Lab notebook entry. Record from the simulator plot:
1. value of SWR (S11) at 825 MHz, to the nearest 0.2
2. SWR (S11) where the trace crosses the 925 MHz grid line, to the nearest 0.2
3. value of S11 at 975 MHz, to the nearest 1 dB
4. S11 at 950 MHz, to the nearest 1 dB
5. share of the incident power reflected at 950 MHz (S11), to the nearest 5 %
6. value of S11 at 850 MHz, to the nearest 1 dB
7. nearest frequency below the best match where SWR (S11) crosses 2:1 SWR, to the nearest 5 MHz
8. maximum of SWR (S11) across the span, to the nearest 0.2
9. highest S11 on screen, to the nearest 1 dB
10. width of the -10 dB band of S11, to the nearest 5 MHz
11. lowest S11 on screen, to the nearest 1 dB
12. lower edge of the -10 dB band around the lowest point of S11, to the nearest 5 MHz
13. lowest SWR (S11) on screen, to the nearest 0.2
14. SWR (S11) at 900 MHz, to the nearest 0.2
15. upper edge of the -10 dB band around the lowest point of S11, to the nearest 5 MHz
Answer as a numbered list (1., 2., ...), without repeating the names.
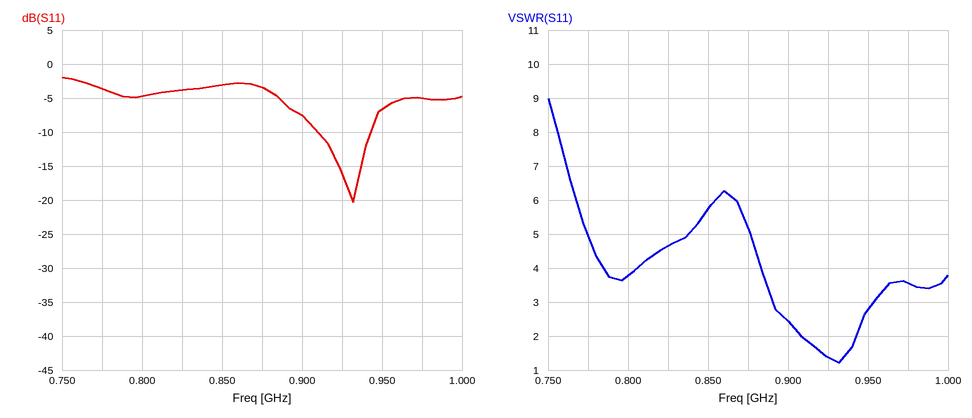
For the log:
1. 4.6
2. 1.4
3. -5 dB
4. -7 dB
5. 20 %
6. -3 dB
7. 910 MHz
8. 9.0
9. -2 dB
10. 35 MHz
11. -20 dB
12. 910 MHz
13. 1.2
14. 2.4
15. 945 MHz
